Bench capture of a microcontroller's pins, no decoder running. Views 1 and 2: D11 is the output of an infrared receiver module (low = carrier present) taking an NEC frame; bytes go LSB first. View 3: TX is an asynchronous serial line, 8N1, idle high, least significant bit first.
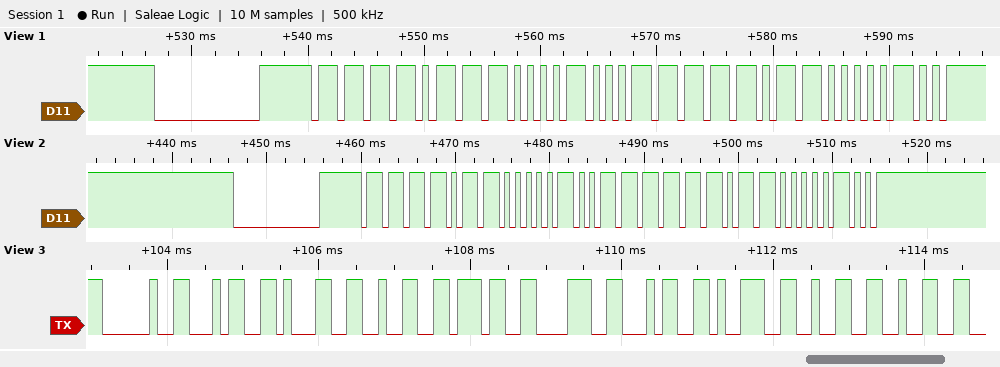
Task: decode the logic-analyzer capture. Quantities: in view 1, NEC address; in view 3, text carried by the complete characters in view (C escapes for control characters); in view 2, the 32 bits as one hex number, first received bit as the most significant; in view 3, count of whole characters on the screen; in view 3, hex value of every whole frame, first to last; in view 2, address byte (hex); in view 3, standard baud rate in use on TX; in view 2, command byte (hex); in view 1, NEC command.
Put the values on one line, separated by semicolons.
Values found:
0xEF; " 412784922"; 0xF609FB04; 10; 0x20 0x34 0x31 0x32 0x37 0x38 0x34 0x39 0x32 0x32; 0x6F; 9600 baud; 0xDF; 0xDF
